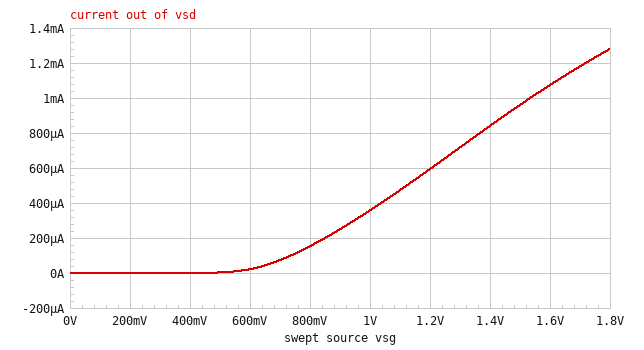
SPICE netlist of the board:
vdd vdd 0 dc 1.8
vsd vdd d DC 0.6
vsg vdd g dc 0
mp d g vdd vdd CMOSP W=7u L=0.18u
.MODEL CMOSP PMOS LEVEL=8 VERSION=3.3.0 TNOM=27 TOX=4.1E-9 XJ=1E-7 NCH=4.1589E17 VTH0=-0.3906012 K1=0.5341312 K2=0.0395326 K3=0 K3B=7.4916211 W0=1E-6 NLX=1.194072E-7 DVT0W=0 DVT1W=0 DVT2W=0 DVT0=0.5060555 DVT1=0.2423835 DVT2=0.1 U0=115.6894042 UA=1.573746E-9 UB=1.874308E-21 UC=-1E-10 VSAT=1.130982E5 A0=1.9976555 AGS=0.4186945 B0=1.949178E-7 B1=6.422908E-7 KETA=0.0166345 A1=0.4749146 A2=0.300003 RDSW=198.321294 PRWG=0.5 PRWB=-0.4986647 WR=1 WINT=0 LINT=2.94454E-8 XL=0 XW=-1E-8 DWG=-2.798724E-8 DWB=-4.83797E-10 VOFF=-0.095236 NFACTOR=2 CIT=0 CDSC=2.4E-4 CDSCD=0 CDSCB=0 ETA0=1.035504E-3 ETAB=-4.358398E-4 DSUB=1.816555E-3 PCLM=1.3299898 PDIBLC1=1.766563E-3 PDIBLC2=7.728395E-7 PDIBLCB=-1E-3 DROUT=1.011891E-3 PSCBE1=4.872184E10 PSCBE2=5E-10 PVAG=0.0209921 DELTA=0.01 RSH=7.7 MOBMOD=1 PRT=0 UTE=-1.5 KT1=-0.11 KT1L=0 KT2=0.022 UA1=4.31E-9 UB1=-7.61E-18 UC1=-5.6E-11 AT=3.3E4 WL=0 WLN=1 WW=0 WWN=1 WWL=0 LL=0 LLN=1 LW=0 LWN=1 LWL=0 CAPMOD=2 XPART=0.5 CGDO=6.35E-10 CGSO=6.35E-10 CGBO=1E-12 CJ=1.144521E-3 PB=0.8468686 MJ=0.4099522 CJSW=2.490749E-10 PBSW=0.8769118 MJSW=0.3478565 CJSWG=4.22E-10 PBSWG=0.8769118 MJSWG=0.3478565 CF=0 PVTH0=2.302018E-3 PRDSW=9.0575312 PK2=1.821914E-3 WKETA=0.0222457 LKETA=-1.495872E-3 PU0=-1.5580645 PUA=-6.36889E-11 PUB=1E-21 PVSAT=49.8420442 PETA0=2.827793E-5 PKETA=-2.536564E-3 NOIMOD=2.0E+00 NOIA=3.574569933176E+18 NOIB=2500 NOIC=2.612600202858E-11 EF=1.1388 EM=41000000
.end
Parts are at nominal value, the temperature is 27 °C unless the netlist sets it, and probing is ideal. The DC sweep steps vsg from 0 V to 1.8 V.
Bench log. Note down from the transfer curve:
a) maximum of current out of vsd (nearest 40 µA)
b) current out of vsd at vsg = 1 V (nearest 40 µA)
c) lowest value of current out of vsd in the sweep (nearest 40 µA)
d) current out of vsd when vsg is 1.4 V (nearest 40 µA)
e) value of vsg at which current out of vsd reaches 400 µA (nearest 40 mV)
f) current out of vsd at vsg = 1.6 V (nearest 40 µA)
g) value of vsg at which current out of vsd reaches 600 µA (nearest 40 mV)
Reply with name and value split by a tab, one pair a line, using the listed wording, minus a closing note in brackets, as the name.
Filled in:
maximum of current out of vsd	1.28 mA
current out of vsd at vsg = 1 V	360 µA
lowest value of current out of vsd in the sweep	0 A
current out of vsd when vsg is 1.4 V	840 µA
value of vsg at which current out of vsd reaches 400 µA	1.04 V
current out of vsd at vsg = 1.6 V	1.08 mA
value of vsg at which current out of vsd reaches 600 µA	1.20 V
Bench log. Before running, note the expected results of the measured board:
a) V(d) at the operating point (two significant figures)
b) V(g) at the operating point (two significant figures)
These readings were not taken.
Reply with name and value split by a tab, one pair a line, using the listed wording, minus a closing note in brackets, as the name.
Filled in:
V(d) at the operating point	1.2 V
V(g) at the operating point	1.8 V
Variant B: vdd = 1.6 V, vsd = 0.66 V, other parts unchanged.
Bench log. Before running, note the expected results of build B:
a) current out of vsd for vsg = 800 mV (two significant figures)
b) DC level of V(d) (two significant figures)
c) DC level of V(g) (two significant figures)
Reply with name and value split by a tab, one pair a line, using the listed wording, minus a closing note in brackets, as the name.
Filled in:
current out of vsd for vsg = 800 mV	160 µA
DC level of V(d)	940 mV
DC level of V(g)	1.6 V
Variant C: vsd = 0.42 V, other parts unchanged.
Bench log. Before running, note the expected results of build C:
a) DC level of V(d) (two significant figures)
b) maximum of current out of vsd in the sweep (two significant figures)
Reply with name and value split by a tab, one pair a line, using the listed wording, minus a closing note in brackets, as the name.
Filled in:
DC level of V(d)	1.4 V
maximum of current out of vsd in the sweep	1.0 mA
